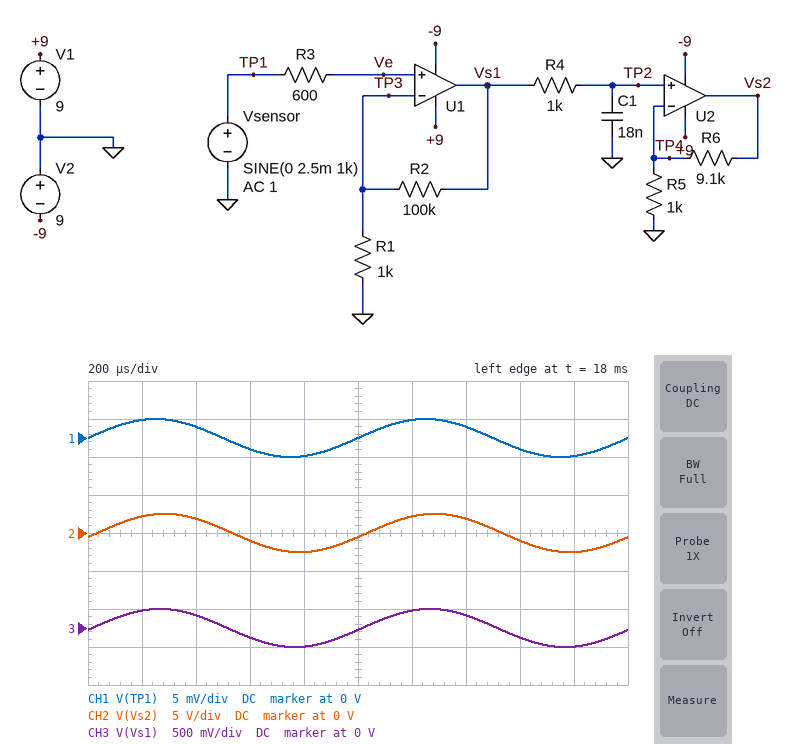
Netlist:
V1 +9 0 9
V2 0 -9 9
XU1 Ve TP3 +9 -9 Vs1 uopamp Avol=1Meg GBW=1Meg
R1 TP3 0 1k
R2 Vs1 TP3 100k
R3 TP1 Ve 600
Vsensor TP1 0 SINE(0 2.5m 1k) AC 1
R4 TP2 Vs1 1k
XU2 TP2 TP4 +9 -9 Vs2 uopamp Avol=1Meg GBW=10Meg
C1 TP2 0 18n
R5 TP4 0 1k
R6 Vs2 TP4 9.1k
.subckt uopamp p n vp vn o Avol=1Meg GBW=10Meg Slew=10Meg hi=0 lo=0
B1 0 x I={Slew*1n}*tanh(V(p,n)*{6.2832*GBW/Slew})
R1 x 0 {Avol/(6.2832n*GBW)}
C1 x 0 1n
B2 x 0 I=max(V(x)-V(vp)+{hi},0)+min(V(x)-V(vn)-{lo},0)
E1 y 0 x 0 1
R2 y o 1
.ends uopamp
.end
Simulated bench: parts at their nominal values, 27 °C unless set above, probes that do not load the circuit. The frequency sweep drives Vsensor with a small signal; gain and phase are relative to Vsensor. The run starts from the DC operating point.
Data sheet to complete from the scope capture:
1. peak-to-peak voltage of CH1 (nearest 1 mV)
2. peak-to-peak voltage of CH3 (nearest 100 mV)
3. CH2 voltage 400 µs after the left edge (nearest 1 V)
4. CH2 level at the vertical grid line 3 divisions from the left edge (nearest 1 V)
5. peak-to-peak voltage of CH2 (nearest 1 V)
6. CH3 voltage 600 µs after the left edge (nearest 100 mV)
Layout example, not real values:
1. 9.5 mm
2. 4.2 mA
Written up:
1. 5 mV
2. 500 mV
3. 2 V
4. -1 V
5. 5 V
6. -100 mV
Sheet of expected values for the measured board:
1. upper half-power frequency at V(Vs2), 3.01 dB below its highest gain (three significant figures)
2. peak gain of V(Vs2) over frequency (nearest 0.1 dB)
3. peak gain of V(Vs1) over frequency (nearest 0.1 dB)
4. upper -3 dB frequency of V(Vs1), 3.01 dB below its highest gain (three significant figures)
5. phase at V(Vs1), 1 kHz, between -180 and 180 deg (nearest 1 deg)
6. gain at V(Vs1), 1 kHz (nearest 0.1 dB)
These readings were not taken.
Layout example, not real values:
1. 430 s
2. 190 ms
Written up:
1. 6.01 kHz
2. 60.2 dB
3. 40.1 dB
4. 9.90 kHz
5. -6 deg
6. 40.0 dB
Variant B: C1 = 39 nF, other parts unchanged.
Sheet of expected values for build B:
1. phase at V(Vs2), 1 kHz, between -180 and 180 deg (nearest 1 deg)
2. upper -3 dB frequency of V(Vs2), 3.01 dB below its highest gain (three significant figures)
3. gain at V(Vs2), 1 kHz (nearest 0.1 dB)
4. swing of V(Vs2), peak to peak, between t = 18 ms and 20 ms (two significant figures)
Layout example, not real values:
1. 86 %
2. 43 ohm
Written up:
1. -20 deg
2. 3.58 kHz
3. 59.9 dB
4. 4.9 V
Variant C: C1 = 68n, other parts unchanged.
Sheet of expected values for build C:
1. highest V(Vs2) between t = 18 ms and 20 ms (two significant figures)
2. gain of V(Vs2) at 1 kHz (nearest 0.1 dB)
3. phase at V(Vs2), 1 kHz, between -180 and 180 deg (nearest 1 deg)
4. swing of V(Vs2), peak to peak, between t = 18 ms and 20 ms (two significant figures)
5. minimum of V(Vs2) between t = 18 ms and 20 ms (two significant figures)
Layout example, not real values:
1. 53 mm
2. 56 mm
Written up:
1. 2.3 V
2. 59.4 dB
3. -29 deg
4. 4.7 V
5. -2.3 V
